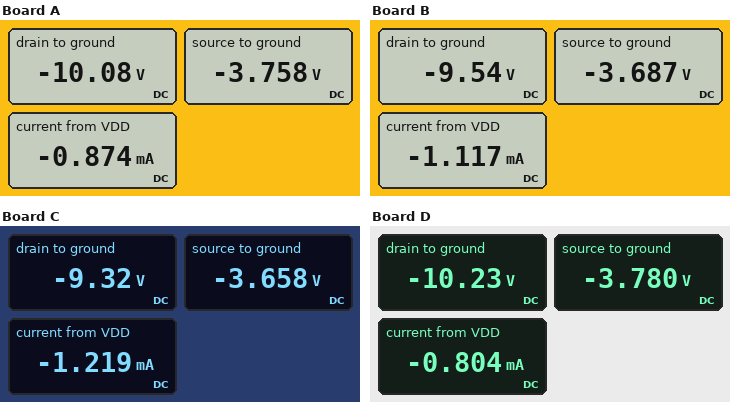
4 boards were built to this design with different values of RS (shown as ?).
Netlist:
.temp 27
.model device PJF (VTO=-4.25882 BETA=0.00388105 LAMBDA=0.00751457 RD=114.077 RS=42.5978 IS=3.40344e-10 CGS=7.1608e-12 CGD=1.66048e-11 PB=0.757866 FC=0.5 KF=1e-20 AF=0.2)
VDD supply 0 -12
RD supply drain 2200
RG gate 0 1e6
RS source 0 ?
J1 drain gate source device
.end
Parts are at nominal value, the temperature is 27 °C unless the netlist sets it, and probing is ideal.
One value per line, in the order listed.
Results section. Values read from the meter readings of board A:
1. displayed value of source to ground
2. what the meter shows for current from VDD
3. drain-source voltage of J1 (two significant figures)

-3.758 V
-0.874 mA
-6.3 V
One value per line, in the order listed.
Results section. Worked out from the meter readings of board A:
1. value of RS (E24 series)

4.3 kΩ
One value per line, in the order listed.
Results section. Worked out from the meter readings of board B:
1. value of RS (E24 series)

3.3 kΩ
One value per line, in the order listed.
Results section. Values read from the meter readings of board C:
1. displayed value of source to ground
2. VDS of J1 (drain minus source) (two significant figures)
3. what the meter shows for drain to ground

-3.658 V
-5.7 V
-9.32 V
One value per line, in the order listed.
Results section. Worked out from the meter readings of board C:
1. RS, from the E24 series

3 kΩ
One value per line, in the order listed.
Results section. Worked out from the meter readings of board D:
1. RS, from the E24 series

4.7 kΩ
